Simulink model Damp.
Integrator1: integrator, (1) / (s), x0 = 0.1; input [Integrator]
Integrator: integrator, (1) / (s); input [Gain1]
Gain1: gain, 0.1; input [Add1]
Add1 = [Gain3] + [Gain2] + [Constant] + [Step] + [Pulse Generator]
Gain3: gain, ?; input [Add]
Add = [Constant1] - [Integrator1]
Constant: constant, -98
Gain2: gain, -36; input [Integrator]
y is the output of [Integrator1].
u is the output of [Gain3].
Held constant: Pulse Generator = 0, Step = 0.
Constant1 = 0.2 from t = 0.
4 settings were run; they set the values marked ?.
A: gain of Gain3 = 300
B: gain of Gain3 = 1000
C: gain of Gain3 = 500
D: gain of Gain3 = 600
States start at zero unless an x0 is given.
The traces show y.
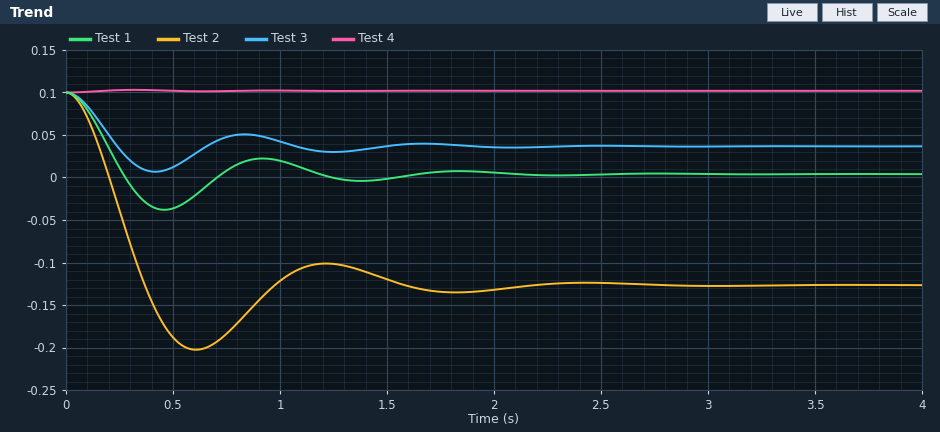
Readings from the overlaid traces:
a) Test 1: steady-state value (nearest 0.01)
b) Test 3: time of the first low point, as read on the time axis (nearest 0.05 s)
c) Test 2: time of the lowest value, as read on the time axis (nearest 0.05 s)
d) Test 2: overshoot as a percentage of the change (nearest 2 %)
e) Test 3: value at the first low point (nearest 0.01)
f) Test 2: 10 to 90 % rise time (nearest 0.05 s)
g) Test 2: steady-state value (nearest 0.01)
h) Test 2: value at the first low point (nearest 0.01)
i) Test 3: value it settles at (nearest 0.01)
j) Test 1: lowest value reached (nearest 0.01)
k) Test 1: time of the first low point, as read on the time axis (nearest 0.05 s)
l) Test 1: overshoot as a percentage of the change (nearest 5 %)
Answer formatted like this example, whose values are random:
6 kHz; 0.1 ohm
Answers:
0.00; 0.40 s; 0.60 s; 34 %; 0.01; 0.25 s; -0.13; -0.20; 0.04; -0.04; 0.45 s; 45 %
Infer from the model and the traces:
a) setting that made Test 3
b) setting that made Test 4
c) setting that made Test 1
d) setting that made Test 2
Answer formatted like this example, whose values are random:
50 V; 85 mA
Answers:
D; B; C; A
